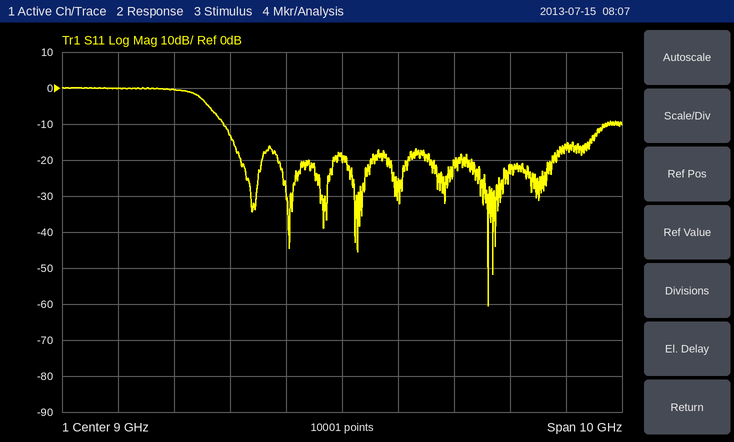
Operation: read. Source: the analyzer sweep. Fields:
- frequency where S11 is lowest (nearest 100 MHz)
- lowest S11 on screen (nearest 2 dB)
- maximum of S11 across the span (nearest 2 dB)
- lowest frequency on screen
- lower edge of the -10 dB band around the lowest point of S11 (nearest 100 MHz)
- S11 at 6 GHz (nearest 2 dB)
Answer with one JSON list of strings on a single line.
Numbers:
["11.6 GHz", "-60 dB", "0 dB", "4 GHz", "6.9 GHz", "0 dB"]
